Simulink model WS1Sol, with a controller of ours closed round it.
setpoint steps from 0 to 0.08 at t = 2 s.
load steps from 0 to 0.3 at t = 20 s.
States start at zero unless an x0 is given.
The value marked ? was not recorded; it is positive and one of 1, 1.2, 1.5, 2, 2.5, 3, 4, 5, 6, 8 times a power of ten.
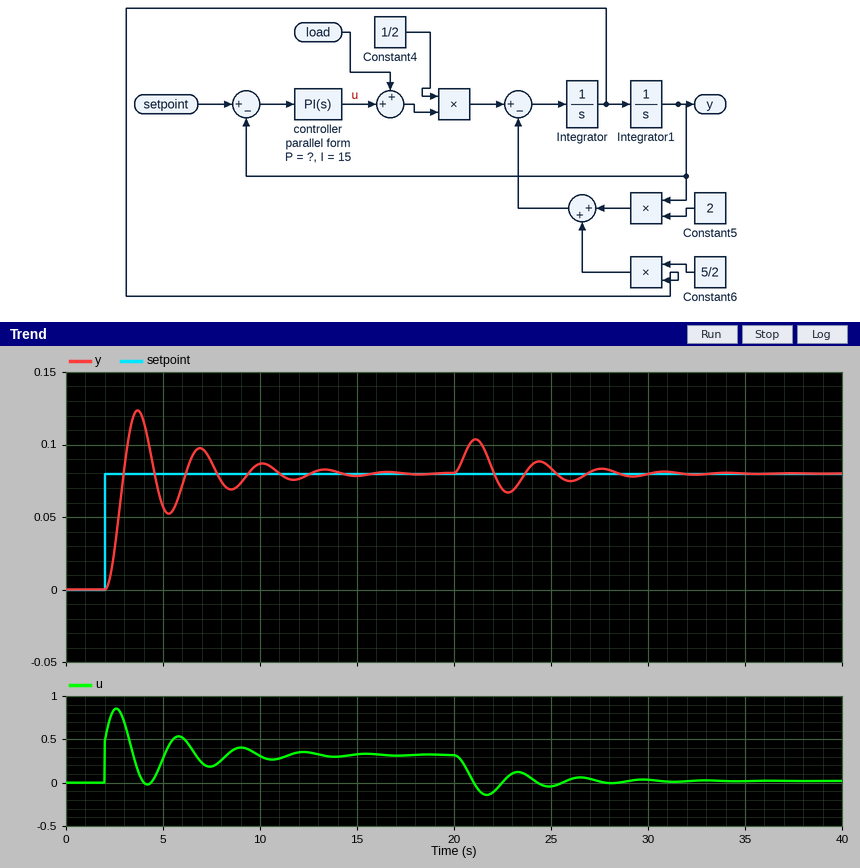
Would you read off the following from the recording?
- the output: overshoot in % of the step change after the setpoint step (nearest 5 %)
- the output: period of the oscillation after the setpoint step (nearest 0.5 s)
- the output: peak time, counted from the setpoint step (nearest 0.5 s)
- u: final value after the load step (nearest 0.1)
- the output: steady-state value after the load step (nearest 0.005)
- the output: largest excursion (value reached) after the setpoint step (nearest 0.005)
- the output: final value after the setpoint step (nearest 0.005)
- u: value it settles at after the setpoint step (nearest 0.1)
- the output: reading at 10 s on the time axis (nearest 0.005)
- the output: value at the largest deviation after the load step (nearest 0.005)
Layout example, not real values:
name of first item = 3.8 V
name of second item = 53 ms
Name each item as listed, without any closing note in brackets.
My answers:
the output: overshoot in % of the step change after the setpoint step = 55 %
the output: period of the oscillation after the setpoint step = 3.0 s
the output: peak time, counted from the setpoint step = 1.5 s
u: final value after the load step = 0.0
the output: steady-state value after the load step = 0.080
the output: largest excursion (value reached) after the setpoint step = 0.125
the output: final value after the setpoint step = 0.080
u: value it settles at after the setpoint step = 0.3
the output: reading at 10 s on the time axis = 0.085
the output: value at the largest deviation after the load step = 0.105
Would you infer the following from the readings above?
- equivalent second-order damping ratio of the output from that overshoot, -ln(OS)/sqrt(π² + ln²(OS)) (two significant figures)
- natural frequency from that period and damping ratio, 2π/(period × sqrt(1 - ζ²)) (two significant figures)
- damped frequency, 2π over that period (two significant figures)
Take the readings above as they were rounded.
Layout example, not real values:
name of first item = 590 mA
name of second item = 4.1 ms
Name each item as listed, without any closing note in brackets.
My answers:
equivalent second-order damping ratio of the output from that overshoot, -ln(OS)/sqrt(π² + ln²(OS)) = 0.19
natural frequency from that period and damping ratio, 2π/(period × sqrt(1 - ζ²)) = 2.1 rad/s
damped frequency, 2π over that period = 2.1 rad/s
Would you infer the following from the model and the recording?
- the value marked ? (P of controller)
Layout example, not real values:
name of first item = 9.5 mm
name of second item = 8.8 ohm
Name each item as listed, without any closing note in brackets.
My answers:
the value marked ? = 6
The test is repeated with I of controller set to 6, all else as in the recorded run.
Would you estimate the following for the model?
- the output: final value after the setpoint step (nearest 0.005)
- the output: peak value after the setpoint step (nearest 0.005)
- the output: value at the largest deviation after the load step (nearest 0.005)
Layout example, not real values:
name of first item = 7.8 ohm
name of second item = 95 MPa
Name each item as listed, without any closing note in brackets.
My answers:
the output: final value after the setpoint step = 0.080
the output: peak value after the setpoint step = 0.090
the output: value at the largest deviation after the load step = 0.110
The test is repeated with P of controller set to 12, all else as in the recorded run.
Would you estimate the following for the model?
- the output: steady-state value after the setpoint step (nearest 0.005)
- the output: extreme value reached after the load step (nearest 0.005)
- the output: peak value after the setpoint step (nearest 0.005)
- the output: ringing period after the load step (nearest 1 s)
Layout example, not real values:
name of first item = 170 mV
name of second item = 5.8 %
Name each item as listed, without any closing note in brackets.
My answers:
the output: steady-state value after the setpoint step = 0.080
the output: extreme value reached after the load step = 0.100
the output: peak value after the setpoint step = 0.110
the output: ringing period after the load step = 3 s
